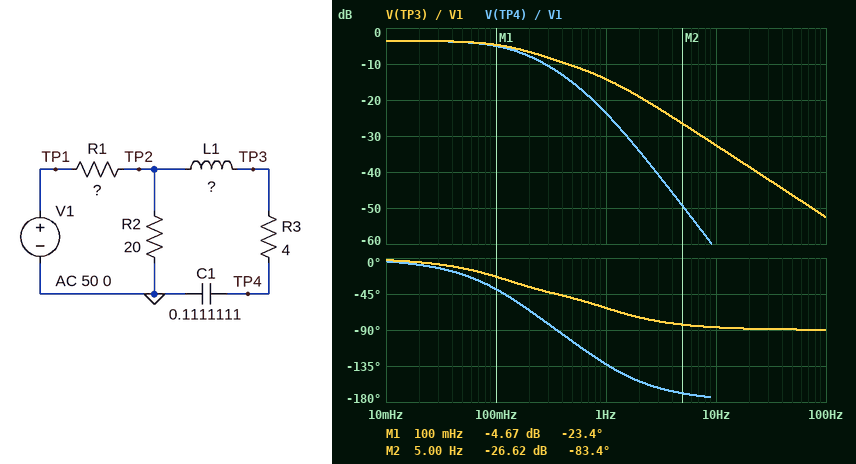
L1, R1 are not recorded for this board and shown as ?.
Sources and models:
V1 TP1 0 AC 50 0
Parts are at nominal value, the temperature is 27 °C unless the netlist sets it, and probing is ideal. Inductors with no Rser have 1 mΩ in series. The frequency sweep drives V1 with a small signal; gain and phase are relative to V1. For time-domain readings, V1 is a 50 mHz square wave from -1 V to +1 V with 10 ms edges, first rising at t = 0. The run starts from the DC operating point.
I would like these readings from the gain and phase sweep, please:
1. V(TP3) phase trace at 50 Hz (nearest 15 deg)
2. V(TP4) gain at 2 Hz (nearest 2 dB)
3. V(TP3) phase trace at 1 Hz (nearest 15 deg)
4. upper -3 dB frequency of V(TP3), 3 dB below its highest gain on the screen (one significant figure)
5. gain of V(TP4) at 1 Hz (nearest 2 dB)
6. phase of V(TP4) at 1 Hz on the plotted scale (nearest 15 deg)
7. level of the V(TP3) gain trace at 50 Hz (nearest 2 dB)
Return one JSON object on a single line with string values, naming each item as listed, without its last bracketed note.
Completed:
{"V(TP3) phase trace at 50 Hz": "-90 deg", "V(TP4) gain at 2 Hz": "-34 dB", "V(TP3) phase trace at 1 Hz": "-60 deg", "upper -3 dB frequency of V(TP3), 3 dB below its highest gain on the screen": "200 mHz", "gain of V(TP4) at 1 Hz": "-24 dB", "phase of V(TP4) at 1 Hz on the plotted scale": "-135 deg", "level of the V(TP3) gain trace at 50 Hz": "-46 dB"}
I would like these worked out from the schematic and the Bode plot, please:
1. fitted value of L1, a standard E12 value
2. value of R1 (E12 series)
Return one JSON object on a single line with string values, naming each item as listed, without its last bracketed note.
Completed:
{"fitted value of L1, a standard E12 value": "1.8 H", "value of R1": "10 Ω"}
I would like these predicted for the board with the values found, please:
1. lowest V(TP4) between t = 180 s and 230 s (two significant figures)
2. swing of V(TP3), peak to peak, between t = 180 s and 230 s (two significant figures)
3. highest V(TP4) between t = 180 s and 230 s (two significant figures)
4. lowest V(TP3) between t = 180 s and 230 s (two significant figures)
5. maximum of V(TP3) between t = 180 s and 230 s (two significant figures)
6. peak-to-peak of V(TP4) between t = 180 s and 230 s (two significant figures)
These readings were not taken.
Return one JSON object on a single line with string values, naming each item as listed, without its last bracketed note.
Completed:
{"lowest V(TP4) between t = 180 s and 230 s": "-670 mV", "swing of V(TP3), peak to peak, between t = 180 s and 230 s": "1.3 V", "highest V(TP4) between t = 180 s and 230 s": "670 mV", "lowest V(TP3) between t = 180 s and 230 s": "-670 mV", "maximum of V(TP3) between t = 180 s and 230 s": "670 mV", "peak-to-peak of V(TP4) between t = 180 s and 230 s": "1.3 V"}
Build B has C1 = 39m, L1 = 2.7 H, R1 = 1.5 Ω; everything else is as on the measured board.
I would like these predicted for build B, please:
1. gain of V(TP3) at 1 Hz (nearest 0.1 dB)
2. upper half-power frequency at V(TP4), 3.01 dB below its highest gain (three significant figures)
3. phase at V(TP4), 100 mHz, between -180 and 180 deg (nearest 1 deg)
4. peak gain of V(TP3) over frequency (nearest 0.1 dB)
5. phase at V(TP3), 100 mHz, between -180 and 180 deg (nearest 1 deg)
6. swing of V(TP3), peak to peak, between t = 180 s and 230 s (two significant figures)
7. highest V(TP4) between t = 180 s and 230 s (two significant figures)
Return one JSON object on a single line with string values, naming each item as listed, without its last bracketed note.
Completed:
{"gain of V(TP3) at 1 Hz": "-8.4 dB", "upper half-power frequency at V(TP4), 3.01 dB below its highest gain": "581 mHz", "phase at V(TP4), 100 mHz, between -180 and 180 deg": "-8 deg", "peak gain of V(TP3) over frequency": "4.4 dB", "phase at V(TP3), 100 mHz, between -180 and 180 deg": "-2 deg", "swing of V(TP3), peak to peak, between t = 180 s and 230 s": "3.3 V", "highest V(TP4) between t = 180 s and 230 s": "1.6 V"}
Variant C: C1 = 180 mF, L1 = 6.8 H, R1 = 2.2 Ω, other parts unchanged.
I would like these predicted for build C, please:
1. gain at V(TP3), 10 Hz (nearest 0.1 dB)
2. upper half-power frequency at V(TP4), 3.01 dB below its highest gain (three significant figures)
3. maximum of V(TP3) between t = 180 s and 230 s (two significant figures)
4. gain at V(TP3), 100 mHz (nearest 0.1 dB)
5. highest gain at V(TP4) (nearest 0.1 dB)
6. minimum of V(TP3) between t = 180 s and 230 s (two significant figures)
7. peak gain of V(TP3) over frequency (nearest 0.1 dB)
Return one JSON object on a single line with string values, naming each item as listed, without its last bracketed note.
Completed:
{"gain at V(TP3), 10 Hz": "-41.5 dB", "upper half-power frequency at V(TP4), 3.01 dB below its highest gain": "169 mHz", "maximum of V(TP3) between t = 180 s and 230 s": "1.3 V", "gain at V(TP3), 100 mHz": "1.3 dB", "highest gain at V(TP4)": "0.5 dB", "minimum of V(TP3) between t = 180 s and 230 s": "-1.3 V", "peak gain of V(TP3) over frequency": "1.5 dB"}
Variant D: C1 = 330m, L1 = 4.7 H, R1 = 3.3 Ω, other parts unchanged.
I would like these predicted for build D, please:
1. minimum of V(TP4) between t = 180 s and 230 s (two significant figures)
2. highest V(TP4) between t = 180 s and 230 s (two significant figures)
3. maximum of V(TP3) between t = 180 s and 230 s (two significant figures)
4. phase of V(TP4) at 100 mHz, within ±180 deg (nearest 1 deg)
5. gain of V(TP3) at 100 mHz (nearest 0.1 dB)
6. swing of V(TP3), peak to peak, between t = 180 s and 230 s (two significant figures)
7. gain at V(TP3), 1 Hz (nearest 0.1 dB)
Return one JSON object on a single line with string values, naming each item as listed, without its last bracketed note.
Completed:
{"minimum of V(TP4) between t = 180 s and 230 s": "-860 mV", "highest V(TP4) between t = 180 s and 230 s": "860 mV", "maximum of V(TP3) between t = 180 s and 230 s": "880 mV", "phase of V(TP4) at 100 mHz, within ±180 deg": "-75 deg", "gain of V(TP3) at 100 mHz": "-2.4 dB", "swing of V(TP3), peak to peak, between t = 180 s and 230 s": "1.8 V", "gain at V(TP3), 1 Hz": "-18.7 dB"}
